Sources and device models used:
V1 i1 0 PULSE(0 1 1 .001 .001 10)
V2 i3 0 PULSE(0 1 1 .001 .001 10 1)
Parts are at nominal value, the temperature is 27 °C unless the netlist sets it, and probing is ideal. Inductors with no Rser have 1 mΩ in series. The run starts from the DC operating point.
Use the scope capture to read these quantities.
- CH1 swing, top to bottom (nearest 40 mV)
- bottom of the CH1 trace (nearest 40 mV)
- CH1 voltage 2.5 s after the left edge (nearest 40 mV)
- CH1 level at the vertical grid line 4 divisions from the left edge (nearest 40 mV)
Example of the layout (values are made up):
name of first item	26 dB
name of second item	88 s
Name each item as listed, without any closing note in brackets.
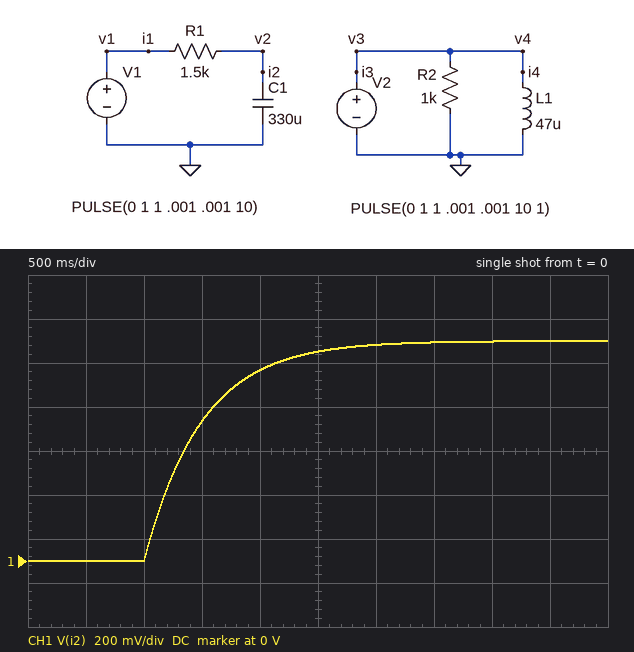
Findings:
CH1 swing, top to bottom	1.00 V
bottom of the CH1 trace	0 V
CH1 voltage 2.5 s after the left edge	960 mV
CH1 level at the vertical grid line 4 divisions from the left edge	880 mV
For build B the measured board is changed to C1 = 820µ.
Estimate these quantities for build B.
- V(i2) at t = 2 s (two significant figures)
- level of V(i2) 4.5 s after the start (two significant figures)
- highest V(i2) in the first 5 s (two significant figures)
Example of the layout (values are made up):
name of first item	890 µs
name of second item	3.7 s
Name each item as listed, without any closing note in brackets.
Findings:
V(i2) at t = 2 s	560 mV
level of V(i2) 4.5 s after the start	940 mV
highest V(i2) in the first 5 s	960 mV
